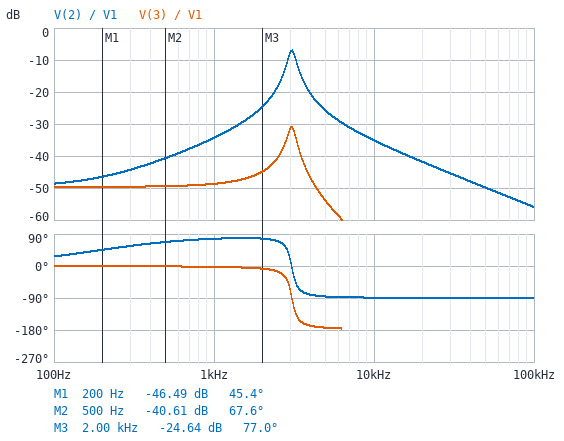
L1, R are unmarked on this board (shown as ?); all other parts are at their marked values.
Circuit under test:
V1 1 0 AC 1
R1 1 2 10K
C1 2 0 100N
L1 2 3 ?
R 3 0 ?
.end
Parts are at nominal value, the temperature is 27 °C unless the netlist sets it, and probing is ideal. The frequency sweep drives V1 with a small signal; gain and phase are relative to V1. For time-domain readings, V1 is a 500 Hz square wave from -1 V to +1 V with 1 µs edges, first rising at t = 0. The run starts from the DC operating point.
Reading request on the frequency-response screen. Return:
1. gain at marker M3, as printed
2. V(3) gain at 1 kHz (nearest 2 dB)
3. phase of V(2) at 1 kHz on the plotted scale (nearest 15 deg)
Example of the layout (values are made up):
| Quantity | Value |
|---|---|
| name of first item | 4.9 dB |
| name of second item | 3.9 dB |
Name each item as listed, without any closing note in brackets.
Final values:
| Quantity | Value |
|---|---|
| gain at marker M3, as printed | -24.64 dB |
| V(3) gain at 1 kHz | -48 dB |
| phase of V(2) at 1 kHz on the plotted scale | 75 deg |
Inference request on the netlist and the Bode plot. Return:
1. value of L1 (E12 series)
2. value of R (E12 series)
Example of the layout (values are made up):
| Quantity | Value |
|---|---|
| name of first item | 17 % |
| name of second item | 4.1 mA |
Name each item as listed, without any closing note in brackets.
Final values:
| Quantity | Value |
|---|---|
| value of L1 | 27 mH |
| value of R | 33 Ω |
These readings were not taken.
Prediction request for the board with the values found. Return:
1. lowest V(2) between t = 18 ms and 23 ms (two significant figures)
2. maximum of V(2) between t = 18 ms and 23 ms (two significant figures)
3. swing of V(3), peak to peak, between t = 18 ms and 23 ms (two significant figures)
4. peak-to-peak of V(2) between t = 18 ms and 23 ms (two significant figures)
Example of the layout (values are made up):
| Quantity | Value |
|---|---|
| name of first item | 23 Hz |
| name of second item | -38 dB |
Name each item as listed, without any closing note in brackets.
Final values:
| Quantity | Value |
|---|---|
| lowest V(2) between t = 18 ms and 23 ms | -75 mV |
| maximum of V(2) between t = 18 ms and 23 ms | 75 mV |
| swing of V(3), peak to peak, between t = 18 ms and 23 ms | 15 mV |
| peak-to-peak of V(2) between t = 18 ms and 23 ms | 150 mV |
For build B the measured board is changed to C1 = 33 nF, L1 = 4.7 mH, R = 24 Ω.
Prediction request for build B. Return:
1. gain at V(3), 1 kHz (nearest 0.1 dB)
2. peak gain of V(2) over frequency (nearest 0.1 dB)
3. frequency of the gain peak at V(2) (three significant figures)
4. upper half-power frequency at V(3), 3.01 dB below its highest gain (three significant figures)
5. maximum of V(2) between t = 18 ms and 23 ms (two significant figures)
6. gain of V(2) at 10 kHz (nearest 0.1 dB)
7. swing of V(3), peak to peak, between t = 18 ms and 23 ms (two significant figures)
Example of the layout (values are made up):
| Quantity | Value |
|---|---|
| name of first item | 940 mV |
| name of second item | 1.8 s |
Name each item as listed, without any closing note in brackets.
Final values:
| Quantity | Value |
|---|---|
| gain at V(3), 1 kHz | -52.4 dB |
| peak gain of V(2) over frequency | -8.6 dB |
| frequency of the gain peak at V(2) | 12.8 kHz |
| upper half-power frequency at V(3), 3.01 dB below its highest gain | 13.4 kHz |
| maximum of V(2) between t = 18 ms and 23 ms | 72 mV |
| gain of V(2) at 10 kHz | -22.6 dB |
| swing of V(3), peak to peak, between t = 18 ms and 23 ms | 13 mV |
